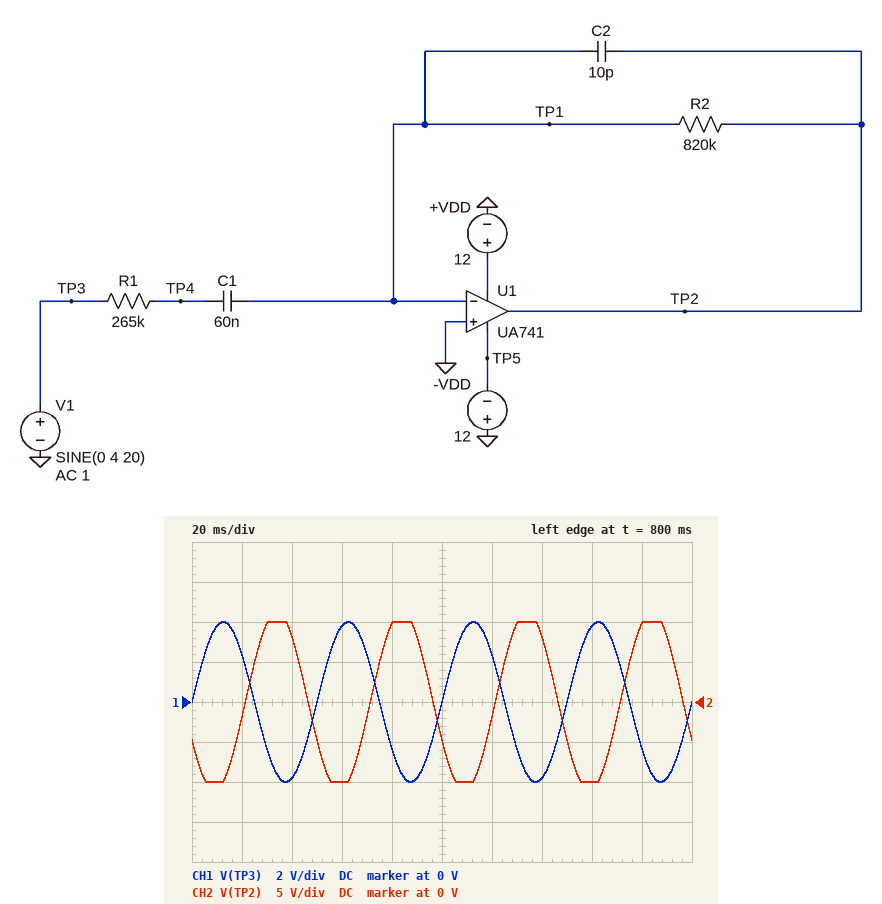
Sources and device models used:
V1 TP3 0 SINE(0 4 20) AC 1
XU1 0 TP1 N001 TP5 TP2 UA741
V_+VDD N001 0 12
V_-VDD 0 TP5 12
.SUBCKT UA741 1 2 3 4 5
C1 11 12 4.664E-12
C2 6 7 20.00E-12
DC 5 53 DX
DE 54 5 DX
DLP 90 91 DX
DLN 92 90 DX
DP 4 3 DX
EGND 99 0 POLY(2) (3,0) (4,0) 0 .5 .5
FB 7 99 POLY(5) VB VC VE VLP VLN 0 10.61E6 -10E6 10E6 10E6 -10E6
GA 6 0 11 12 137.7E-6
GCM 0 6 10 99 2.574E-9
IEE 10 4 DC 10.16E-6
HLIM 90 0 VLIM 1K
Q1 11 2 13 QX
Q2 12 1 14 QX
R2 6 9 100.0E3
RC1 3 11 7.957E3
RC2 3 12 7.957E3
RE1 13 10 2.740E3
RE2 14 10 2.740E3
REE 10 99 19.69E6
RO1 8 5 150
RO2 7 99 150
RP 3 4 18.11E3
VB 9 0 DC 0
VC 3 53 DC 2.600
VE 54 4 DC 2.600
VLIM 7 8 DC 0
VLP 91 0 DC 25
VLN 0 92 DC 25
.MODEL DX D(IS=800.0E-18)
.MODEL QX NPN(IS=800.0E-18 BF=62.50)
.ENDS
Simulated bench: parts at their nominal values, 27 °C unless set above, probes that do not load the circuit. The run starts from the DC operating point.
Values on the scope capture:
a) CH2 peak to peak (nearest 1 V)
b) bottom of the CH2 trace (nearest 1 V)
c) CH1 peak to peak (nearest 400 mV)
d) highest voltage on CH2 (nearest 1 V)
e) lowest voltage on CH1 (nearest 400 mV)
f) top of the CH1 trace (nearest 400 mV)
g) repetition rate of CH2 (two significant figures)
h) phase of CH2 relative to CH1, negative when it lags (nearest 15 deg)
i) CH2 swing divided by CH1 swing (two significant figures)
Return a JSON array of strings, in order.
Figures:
["20 V", "-10 V", "8.0 V", "10 V", "-4.0 V", "4.0 V", "20 Hz", "-150 deg", "2.5"]
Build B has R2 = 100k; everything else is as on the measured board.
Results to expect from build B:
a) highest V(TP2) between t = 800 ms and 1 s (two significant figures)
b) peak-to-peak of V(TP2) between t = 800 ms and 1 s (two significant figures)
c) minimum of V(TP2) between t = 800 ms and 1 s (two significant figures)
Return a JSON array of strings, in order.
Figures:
["1.4 V", "2.7 V", "-1.3 V"]
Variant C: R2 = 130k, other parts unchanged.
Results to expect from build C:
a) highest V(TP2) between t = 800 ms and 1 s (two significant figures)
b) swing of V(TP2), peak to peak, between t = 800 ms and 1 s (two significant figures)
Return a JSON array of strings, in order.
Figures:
["1.8 V", "3.5 V"]
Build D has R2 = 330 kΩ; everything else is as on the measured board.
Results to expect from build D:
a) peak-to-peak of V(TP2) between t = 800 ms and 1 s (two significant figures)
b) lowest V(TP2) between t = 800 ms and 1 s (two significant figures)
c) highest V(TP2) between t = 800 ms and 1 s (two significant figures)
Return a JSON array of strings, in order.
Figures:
["8.9 V", "-4.4 V", "4.5 V"]
